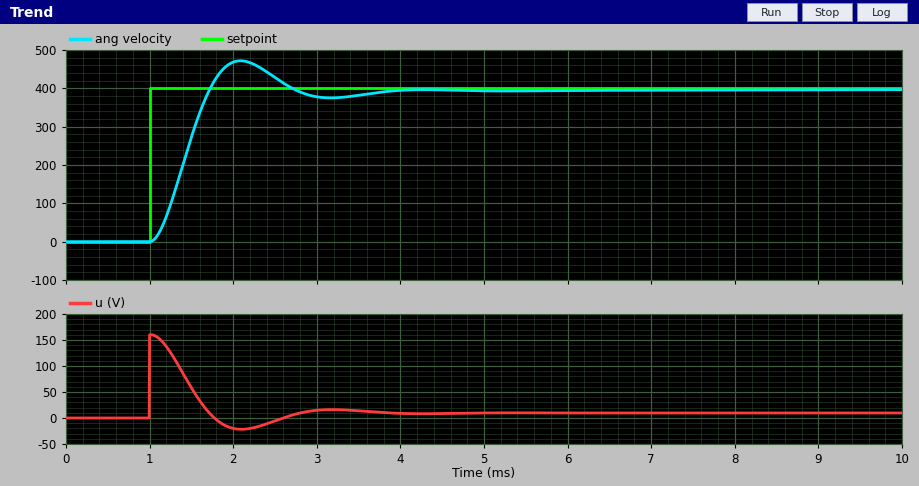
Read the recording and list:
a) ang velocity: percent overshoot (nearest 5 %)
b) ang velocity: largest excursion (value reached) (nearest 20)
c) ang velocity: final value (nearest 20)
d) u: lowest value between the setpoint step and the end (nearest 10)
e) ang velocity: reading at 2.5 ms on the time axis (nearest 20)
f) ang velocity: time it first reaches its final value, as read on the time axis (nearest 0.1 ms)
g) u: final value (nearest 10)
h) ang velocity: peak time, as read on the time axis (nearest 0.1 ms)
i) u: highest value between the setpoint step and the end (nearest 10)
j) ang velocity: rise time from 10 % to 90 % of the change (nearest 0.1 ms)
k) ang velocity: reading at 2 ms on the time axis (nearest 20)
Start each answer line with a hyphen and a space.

- 20 %
- 480
- 400
- -20
- 420
- 1.7 ms
- 10
- 2.1 ms
- 160
- 0.5 ms
- 460
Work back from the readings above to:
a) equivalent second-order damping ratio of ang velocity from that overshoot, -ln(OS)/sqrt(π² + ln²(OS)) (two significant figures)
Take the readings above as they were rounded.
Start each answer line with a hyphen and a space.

- 0.46
